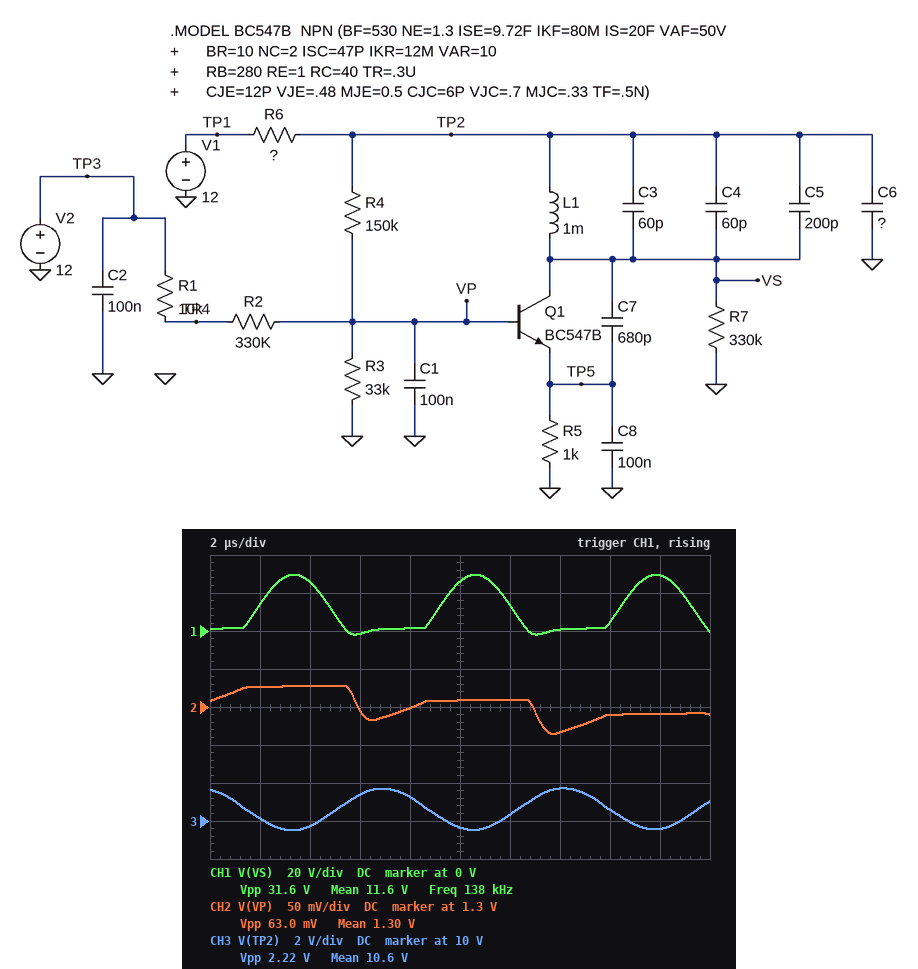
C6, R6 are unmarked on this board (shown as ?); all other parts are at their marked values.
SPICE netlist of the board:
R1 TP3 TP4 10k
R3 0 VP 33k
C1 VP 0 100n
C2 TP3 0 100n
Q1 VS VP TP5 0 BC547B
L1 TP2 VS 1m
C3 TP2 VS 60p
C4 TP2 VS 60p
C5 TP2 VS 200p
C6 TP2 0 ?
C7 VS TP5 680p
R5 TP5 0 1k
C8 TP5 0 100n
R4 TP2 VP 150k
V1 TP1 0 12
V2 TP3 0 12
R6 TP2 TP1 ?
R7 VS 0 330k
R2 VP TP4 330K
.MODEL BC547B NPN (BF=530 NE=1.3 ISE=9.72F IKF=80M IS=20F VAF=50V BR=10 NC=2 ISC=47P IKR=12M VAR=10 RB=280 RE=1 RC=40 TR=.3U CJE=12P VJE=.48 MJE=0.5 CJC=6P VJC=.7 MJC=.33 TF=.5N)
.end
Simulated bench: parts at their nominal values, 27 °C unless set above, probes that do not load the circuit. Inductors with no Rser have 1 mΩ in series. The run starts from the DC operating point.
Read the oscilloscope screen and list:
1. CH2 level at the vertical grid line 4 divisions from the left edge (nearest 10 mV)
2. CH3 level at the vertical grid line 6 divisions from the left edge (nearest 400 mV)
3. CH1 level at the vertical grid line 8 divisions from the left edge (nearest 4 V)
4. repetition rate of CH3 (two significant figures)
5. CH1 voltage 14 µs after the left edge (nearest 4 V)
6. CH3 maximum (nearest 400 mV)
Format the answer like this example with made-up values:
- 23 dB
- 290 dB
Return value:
- 1.30 V
- 10.4 V
- 4 V
- 140 kHz
- 0 V
- 11.6 V
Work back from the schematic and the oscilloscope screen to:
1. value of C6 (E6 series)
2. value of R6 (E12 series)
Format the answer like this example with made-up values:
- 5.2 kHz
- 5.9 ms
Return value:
- 15 nF
- 2.2 kΩ
